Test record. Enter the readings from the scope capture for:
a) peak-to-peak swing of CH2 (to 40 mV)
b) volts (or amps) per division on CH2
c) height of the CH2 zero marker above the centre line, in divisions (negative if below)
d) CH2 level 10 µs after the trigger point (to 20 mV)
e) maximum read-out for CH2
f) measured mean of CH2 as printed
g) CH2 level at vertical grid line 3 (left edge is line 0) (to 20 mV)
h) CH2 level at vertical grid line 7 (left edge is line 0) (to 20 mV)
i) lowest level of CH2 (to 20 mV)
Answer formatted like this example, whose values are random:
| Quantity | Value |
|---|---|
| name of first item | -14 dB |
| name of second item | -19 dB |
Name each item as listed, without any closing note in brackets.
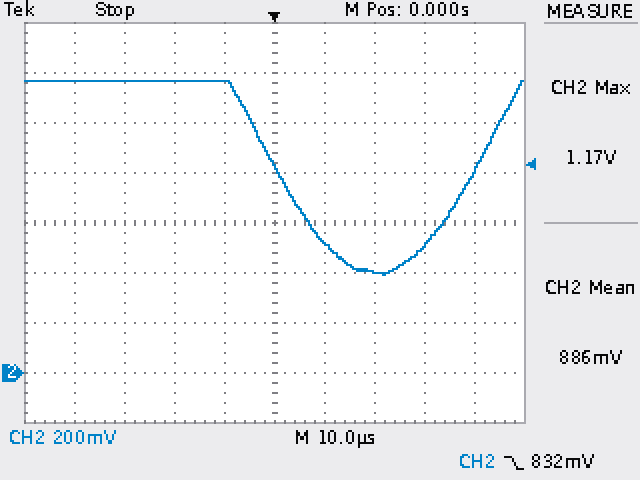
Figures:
| Quantity | Value |
|---|---|
| peak-to-peak swing of CH2 | 760 mV |
| volts (or amps) per division on CH2 | 200 mV |
| height of the CH2 zero marker above the centre line, in divisions | -3.0 div |
| CH2 level 10 µs after the trigger point | 520 mV |
| maximum read-out for CH2 | 1.17 V |
| measured mean of CH2 as printed | 886 mV |
| CH2 level at vertical grid line 3 (left edge is line 0) | 1.16 V |
| CH2 level at vertical grid line 7 (left edge is line 0) | 400 mV |
| lowest level of CH2 | 400 mV |
